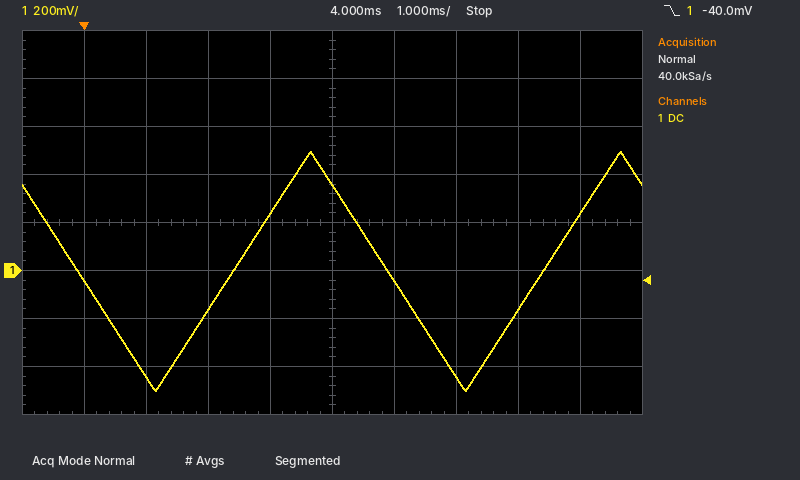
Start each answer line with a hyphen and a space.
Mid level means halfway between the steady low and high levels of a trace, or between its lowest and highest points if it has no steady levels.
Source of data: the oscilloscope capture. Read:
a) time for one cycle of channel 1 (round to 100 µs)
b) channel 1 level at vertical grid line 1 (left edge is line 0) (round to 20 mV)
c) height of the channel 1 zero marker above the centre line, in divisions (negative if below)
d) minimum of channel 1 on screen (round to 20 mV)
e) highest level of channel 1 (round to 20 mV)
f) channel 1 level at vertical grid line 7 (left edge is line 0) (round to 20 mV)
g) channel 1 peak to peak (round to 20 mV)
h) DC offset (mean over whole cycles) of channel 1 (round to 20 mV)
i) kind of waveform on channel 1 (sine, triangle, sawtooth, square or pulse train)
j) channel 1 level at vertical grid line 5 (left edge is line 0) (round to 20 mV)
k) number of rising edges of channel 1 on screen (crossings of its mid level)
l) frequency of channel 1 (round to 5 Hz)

- 5.0 ms
- -40 mV
- -1.0 div
- -500 mV
- 500 mV
- -440 mV
- 1.00 V
- 0 mV
- triangle
- 360 mV
- 2
- 200 Hz
